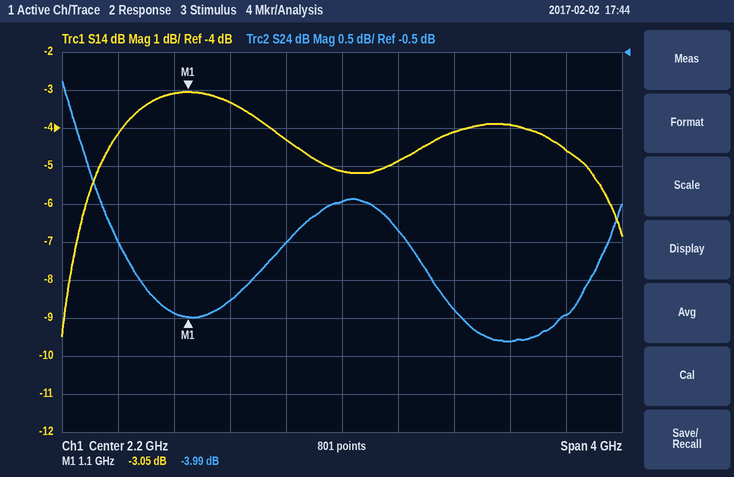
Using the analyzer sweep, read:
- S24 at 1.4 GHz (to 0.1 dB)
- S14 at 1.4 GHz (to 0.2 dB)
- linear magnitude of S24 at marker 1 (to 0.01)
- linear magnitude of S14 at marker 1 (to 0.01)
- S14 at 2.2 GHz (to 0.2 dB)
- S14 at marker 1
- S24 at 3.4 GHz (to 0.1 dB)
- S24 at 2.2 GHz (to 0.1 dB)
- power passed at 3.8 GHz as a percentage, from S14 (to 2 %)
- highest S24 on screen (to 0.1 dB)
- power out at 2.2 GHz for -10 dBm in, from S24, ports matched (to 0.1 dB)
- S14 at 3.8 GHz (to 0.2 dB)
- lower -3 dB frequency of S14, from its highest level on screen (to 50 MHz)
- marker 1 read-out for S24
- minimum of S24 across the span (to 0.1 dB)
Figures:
-3.8 dB
-3.4 dB
0.63
0.70
-5.2 dB
-3.05 dB
-4.3 dB
-2.5 dB
34 %
-0.9 dB
-12.5 dBm
-4.6 dB
350 MHz
-3.99 dB
-4.3 dB
